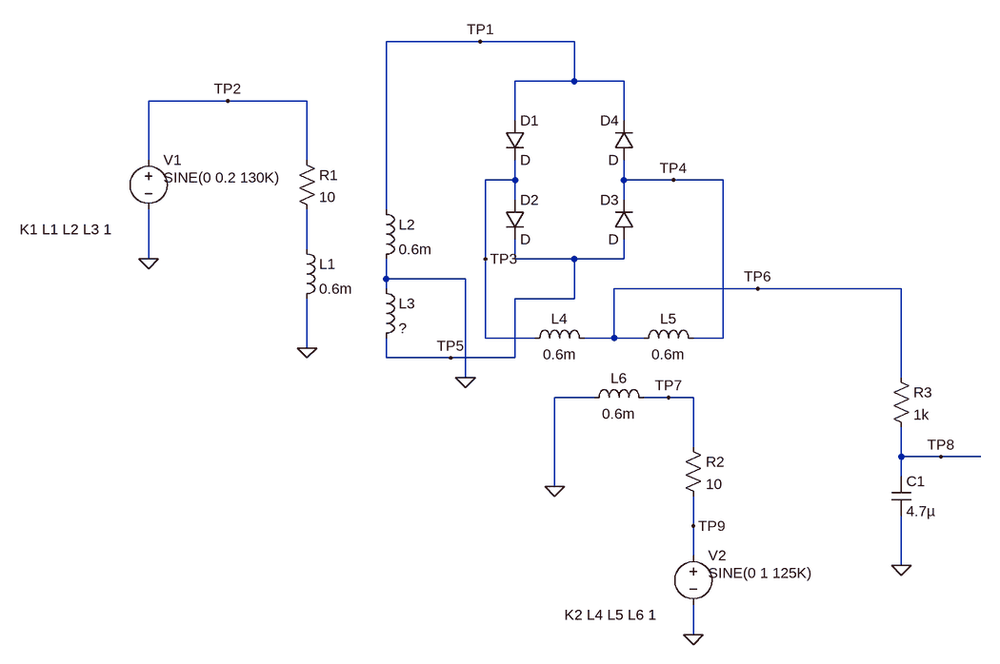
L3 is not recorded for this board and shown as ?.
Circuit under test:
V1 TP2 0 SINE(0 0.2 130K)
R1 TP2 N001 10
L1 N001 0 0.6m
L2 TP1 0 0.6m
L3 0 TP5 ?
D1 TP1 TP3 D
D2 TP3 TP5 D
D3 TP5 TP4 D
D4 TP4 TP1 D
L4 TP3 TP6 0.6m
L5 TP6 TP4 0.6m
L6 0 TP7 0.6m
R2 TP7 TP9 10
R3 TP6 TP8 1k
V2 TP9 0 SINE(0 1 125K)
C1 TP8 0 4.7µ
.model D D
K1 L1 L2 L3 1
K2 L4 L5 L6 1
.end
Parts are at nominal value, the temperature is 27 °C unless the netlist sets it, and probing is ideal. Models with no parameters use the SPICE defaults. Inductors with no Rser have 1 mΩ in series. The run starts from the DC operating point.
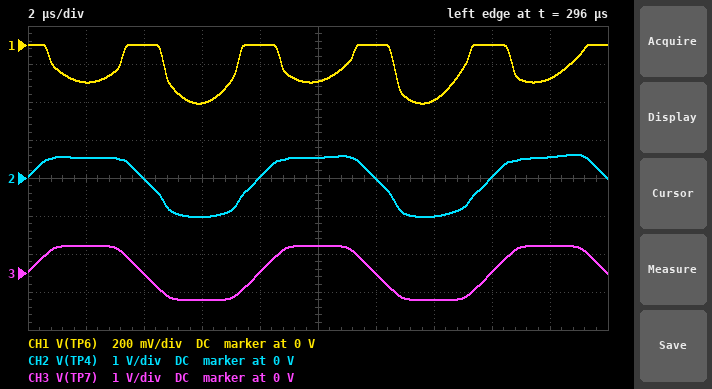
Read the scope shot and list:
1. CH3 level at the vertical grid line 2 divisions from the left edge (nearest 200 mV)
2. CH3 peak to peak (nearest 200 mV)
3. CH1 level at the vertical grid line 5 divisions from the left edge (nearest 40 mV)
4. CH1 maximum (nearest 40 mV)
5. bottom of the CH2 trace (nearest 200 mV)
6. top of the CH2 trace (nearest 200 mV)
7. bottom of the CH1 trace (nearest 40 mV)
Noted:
0 V
1.4 V
-200 mV
0 V
-1.0 V
600 mV
-320 mV
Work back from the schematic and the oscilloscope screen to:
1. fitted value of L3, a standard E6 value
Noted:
1.5 mH
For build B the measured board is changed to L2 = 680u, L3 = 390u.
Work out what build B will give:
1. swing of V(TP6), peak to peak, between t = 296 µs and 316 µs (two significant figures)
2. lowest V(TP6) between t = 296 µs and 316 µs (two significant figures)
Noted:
210 mV
-210 mV
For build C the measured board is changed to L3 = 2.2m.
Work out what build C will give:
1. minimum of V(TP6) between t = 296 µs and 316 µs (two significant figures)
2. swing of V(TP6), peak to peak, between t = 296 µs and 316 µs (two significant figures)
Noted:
-370 mV
370 mV
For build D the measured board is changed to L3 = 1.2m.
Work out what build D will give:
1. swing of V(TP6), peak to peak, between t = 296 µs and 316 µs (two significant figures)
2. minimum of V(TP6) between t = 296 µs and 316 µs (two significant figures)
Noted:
280 mV
-280 mV
